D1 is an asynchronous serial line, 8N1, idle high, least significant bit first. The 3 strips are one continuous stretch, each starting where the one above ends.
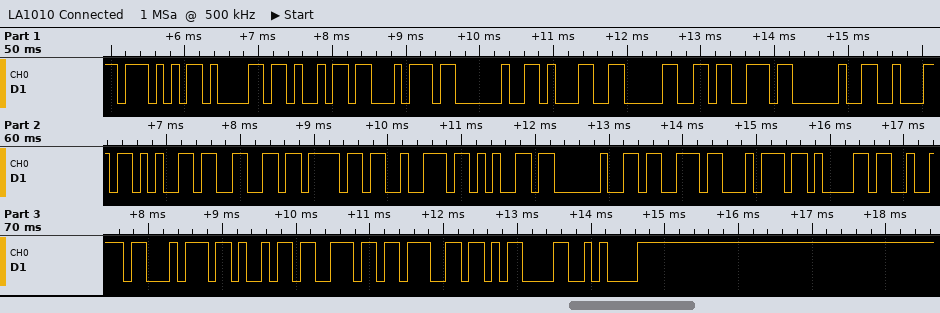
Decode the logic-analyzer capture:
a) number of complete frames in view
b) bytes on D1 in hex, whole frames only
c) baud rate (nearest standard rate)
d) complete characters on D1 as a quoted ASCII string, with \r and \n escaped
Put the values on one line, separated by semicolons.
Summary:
26; 57 61 69 74 20 31 30 73 20 62 65 66 6F 72 65 20 73 74 61 72 74 69 6E 67 0D 0A; 9600 baud; "Wait 10s before starting\r\n"
